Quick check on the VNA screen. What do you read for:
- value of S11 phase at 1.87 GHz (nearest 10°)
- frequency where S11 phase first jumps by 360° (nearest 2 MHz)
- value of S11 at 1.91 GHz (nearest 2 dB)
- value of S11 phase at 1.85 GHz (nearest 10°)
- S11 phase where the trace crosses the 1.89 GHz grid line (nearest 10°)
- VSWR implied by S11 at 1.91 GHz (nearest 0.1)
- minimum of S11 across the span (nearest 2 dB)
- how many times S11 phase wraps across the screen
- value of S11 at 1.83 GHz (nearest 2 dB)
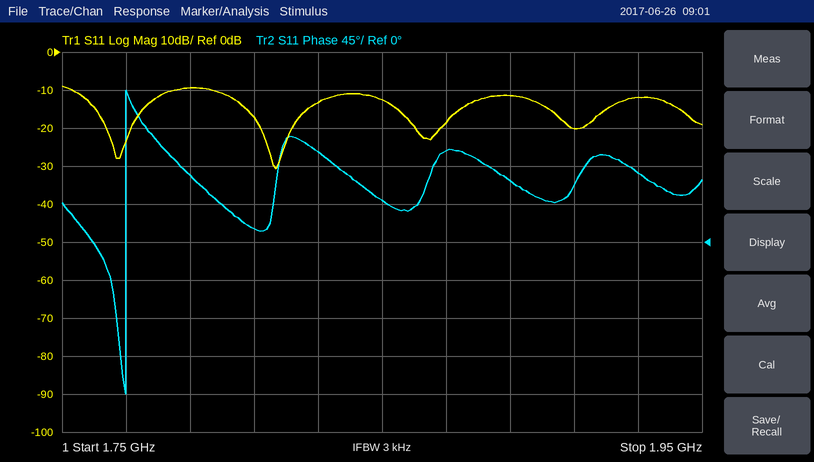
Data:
110°
1.770 GHz
-20 dB
50°
70°
1.2
-30 dB
1
-14 dB
